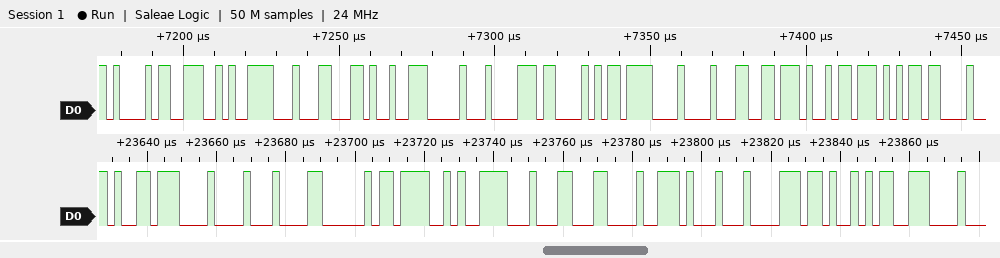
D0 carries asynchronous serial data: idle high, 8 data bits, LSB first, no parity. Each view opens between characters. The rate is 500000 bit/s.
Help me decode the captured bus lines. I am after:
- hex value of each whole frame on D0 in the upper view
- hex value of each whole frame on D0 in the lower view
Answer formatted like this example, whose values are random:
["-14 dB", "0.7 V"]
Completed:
["A1, 4E, 1E, 8C, C9, 10, B8, A8, 0F, 88, 76, DA, B5", "D9, 08, 84, A0, 4F, 1E, 8C, C8, 11, B8, A9, 0E"]
